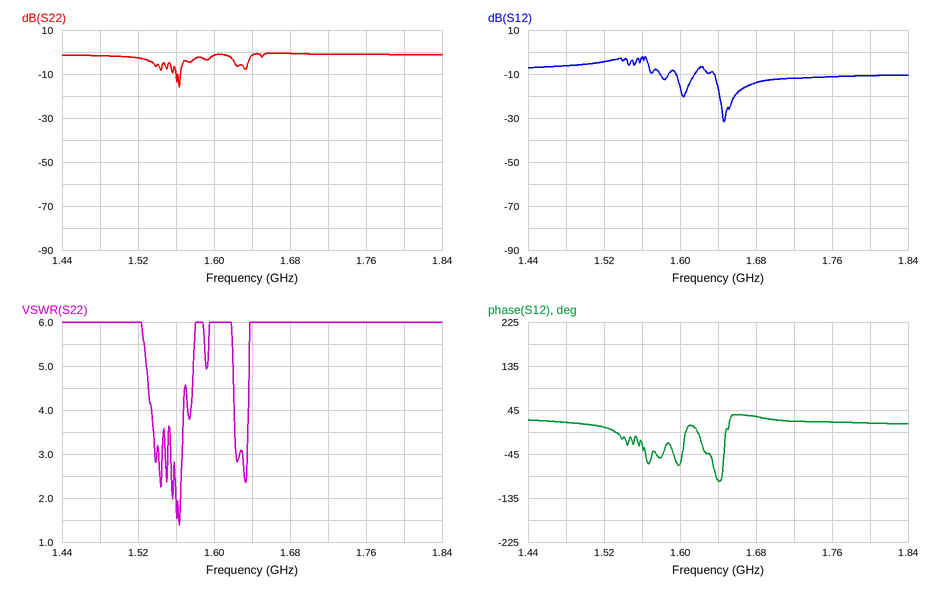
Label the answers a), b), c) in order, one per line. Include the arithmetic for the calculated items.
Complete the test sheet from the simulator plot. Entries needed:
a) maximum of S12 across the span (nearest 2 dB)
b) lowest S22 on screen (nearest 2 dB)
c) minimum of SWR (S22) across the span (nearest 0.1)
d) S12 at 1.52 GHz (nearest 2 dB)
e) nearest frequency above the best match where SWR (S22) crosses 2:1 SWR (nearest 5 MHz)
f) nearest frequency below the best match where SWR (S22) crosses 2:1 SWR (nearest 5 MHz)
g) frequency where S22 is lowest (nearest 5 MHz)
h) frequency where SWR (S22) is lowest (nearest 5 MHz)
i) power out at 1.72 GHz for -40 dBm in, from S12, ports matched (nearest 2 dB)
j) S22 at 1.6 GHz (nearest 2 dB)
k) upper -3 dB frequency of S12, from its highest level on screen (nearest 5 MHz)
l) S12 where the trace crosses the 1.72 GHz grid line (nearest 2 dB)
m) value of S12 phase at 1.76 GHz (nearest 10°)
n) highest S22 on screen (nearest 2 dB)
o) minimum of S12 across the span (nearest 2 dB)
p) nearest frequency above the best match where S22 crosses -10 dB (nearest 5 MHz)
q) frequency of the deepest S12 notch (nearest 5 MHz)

a) -2 dB
b) -16 dB
c) 1.4
d) -4 dB
e) 1.565 GHz
f) 1.560 GHz
g) 1.565 GHz
h) 1.565 GHz
i) -40 dBm + (-12 dB) = -52 dBm
j) -2 dB
k) 1.565 GHz
l) -12 dB
m) 20°
n) 0 dB
o) -32 dB
p) 1.565 GHz
q) 1.645 GHz
